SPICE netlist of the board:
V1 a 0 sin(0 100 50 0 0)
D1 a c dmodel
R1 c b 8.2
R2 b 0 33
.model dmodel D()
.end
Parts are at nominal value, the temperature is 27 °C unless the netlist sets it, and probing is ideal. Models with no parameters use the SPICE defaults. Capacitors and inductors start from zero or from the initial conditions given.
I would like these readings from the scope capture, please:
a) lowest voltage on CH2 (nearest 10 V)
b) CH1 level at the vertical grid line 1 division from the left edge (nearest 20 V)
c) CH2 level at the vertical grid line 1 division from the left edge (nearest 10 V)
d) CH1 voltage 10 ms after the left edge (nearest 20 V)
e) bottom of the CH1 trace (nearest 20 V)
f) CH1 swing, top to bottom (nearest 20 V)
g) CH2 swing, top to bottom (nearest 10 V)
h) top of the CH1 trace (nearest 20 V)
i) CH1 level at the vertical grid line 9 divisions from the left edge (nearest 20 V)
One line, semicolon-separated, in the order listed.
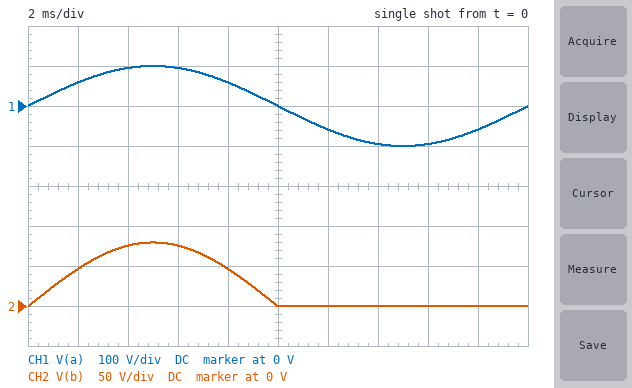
0 V; 60 V; 50 V; 0 V; -100 V; 200 V; 80 V; 100 V; -60 V
